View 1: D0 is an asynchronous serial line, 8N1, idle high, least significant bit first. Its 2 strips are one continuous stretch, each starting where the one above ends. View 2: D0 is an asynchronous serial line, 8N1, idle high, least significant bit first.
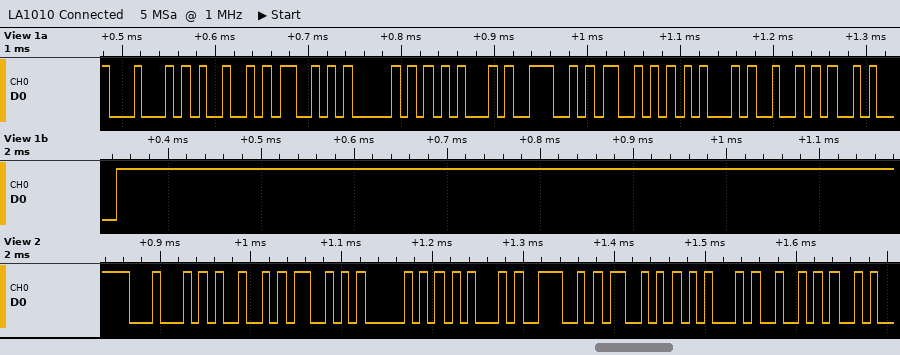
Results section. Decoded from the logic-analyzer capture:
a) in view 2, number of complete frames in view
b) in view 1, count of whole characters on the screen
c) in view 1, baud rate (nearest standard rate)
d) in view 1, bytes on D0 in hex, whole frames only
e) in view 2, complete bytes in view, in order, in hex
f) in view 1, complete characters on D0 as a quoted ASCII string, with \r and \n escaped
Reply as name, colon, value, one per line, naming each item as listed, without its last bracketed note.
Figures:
in view 2, number of complete frames in view: 9
in view 1, count of whole characters on the screen: 10
in view 1, baud rate: 115200 baud
in view 1, bytes on D0 in hex, whole frames only: 44 49 53 50 45 4E 53 45 52 0A
in view 2, complete bytes in view, in order, in hex: 44 49 53 50 45 4E 53 45 52
in view 1, complete characters on D0 as a quoted ASCII string, with \r and \n escaped: "DISPENSER\n"
